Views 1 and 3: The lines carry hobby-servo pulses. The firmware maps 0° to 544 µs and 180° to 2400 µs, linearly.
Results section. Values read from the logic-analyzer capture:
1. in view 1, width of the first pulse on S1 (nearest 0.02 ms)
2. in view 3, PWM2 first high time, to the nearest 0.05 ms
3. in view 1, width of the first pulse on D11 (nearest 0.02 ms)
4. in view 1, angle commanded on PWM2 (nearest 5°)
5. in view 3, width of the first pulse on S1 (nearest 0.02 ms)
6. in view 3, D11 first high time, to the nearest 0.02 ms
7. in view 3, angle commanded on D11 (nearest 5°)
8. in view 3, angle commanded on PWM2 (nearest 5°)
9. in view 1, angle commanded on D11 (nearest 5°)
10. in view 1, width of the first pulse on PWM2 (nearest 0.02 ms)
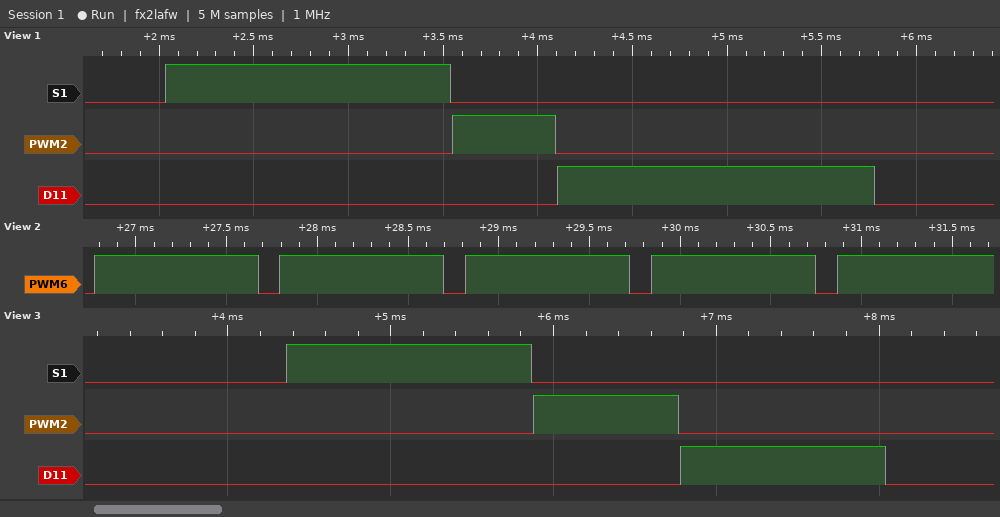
1.50 ms
0.90 ms
1.68 ms
0°
1.50 ms
1.26 ms
70°
35°
110°
0.54 ms
